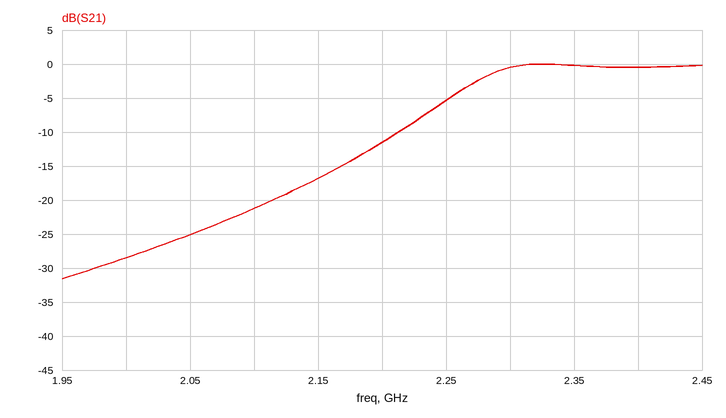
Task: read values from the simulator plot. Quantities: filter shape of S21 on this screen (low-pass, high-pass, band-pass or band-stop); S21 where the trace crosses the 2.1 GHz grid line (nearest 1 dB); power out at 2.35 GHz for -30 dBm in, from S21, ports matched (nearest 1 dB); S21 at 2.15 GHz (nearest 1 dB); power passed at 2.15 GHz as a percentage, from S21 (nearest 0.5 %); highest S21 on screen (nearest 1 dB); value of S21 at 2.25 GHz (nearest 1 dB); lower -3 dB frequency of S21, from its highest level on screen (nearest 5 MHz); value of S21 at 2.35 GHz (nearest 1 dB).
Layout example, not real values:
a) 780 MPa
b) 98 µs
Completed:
a) high-pass
b) -21 dB
c) -30 dBm
d) -17 dB
e) 2.0 %
f) 0 dB
g) -5 dB
h) 2.270 GHz
i) 0 dB
